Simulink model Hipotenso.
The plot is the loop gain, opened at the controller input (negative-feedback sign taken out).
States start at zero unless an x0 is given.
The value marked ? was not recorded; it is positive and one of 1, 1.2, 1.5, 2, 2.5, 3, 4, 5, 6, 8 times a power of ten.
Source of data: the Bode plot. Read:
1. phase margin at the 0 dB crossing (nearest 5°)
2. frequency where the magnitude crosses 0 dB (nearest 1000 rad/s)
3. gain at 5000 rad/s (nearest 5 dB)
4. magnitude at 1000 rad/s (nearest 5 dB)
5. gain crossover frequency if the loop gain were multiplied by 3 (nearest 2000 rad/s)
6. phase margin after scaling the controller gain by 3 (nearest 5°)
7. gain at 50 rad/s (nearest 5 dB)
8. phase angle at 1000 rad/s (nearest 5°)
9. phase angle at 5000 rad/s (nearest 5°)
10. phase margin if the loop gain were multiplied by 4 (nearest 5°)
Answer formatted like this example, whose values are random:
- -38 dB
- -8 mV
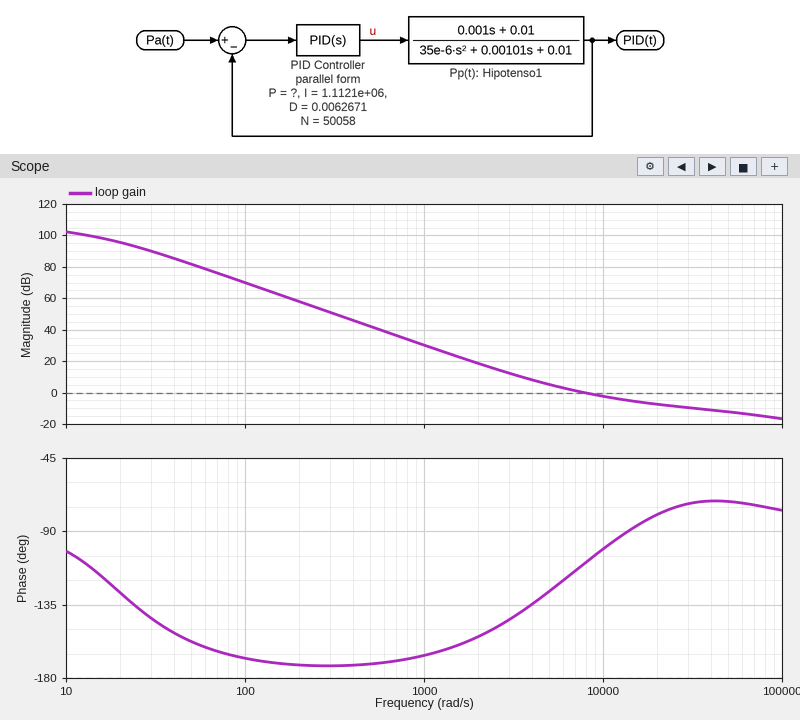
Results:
- 70°
- 8000 rad/s
- 5 dB
- 30 dB
- 30000 rad/s
- 105°
- 80 dB
- -165°
- -125°
- 110°
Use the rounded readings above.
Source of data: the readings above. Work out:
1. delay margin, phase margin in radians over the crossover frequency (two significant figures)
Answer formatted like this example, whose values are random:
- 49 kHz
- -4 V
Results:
- 0.00015 s
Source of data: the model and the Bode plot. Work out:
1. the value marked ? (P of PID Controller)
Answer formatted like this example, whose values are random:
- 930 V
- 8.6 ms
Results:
- 250
